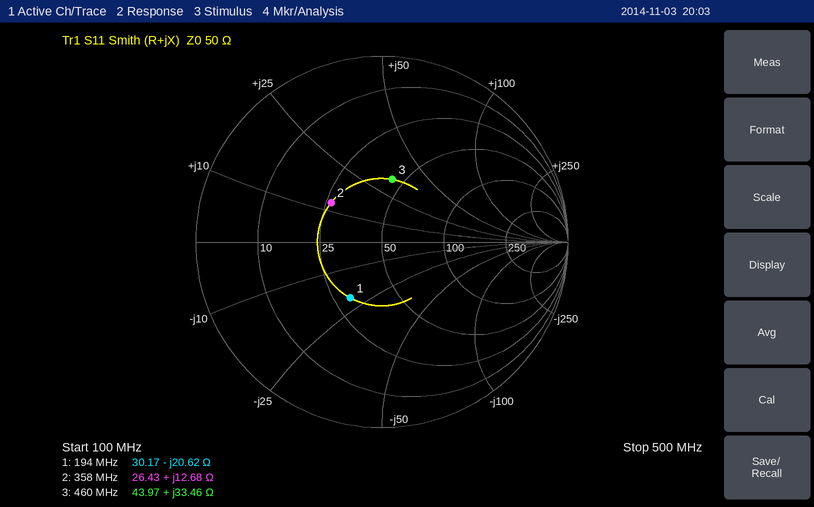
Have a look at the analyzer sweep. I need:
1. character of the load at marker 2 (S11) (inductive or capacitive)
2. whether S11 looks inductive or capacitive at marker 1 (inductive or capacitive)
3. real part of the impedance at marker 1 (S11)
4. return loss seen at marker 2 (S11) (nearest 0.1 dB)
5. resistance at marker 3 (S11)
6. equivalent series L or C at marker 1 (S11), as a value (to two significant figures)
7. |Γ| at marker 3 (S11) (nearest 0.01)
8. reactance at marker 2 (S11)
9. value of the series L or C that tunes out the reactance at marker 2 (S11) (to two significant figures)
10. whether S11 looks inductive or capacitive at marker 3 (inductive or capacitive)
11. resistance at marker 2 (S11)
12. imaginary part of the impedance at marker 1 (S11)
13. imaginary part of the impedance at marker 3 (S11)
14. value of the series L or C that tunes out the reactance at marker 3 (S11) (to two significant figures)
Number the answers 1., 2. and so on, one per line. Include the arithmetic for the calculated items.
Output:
1. inductive
2. capacitive
3. 30.17 Ω
4. 9.2 dB
5. 43.97 Ω
6. C = 1/(2π × 194 MHz × 20.62 Ω) ≈ 40 pF
7. 0.34
8. +12.68 Ω
9. C = 1/(2π × 358 MHz × 12.68 Ω) ≈ 35 pF
10. inductive
11. 26.43 Ω
12. -20.62 Ω
13. +33.46 Ω
14. C = 1/(2π × 460 MHz × 33.46 Ω) ≈ 10 pF
